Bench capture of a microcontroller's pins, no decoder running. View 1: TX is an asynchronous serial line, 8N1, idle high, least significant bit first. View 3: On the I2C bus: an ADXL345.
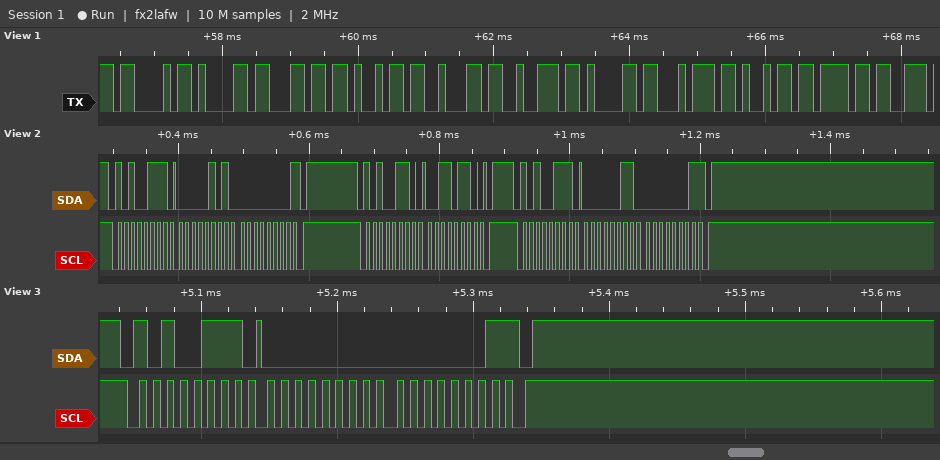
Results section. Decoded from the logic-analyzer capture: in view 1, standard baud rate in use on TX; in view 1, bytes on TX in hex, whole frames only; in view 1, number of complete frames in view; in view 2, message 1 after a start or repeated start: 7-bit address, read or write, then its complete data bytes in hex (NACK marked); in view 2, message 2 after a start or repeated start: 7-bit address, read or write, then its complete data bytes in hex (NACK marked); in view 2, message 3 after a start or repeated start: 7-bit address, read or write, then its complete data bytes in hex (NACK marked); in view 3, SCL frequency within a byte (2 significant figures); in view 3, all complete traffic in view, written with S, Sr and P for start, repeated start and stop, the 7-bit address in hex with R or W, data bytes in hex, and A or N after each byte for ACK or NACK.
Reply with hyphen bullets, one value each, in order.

- 9600 baud
- 43 61 6C 69 62 72 61 74 69 6F
- 10
- 0x53 read: 05 00 NACK
- 0x53 write: 36
- 0x53 read: 03 01 NACK
- 100 kHz
- S 53R A 00 A 01 N P
